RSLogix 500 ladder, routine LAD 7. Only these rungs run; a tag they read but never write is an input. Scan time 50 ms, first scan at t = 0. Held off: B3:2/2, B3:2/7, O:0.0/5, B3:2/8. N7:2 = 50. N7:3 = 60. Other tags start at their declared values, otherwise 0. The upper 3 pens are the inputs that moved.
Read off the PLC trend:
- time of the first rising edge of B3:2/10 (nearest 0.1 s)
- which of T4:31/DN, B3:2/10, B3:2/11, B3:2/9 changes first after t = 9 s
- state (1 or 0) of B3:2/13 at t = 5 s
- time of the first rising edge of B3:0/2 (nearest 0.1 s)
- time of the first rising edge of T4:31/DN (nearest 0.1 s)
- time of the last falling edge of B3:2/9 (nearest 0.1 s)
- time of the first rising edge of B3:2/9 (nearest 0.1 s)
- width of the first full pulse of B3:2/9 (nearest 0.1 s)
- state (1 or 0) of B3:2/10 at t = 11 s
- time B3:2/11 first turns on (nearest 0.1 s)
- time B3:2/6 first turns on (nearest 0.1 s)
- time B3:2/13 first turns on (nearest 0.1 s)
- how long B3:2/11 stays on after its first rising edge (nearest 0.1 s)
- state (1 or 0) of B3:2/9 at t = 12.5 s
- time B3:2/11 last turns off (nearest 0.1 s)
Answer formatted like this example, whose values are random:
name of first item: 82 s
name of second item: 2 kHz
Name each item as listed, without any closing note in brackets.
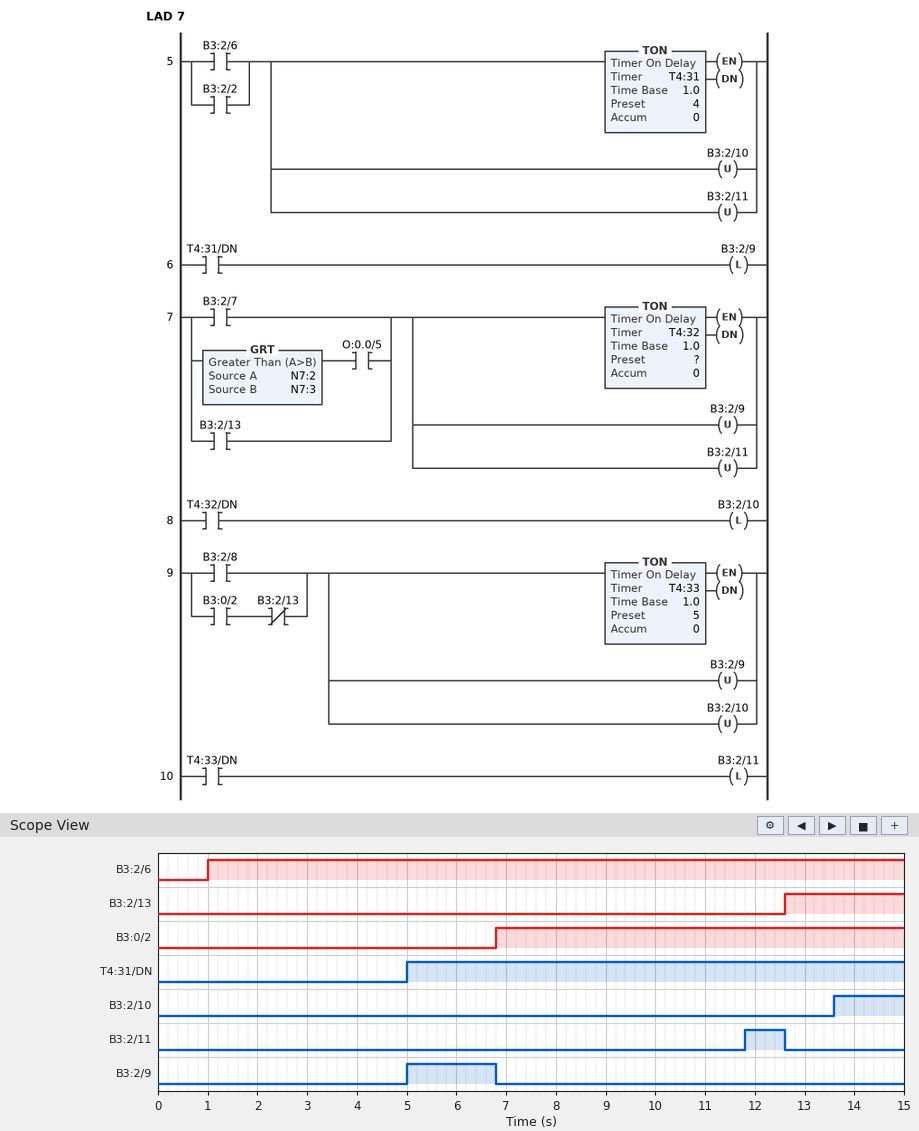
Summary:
time of the first rising edge of B3:2/10: 13.6 s
which of T4:31/DN, B3:2/10, B3:2/11, B3:2/9 changes first after t = 9 s: B3:2/11
state (1 or 0) of B3:2/13 at t = 5 s: 0
time of the first rising edge of B3:0/2: 6.8 s
time of the first rising edge of T4:31/DN: 5.0 s
time of the last falling edge of B3:2/9: 6.8 s
time of the first rising edge of B3:2/9: 5.0 s
width of the first full pulse of B3:2/9: 1.8 s
state (1 or 0) of B3:2/10 at t = 11 s: 0
time B3:2/11 first turns on: 11.8 s
time B3:2/6 first turns on: 1.0 s
time B3:2/13 first turns on: 12.6 s
how long B3:2/11 stays on after its first rising edge: 0.8 s
state (1 or 0) of B3:2/9 at t = 12.5 s: 0
time B3:2/11 last turns off: 12.6 s
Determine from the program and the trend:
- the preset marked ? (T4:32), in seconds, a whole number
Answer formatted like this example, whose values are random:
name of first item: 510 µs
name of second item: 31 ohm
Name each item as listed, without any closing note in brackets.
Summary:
the preset marked ? (T4:32), in seconds, a whole number: 1 s
